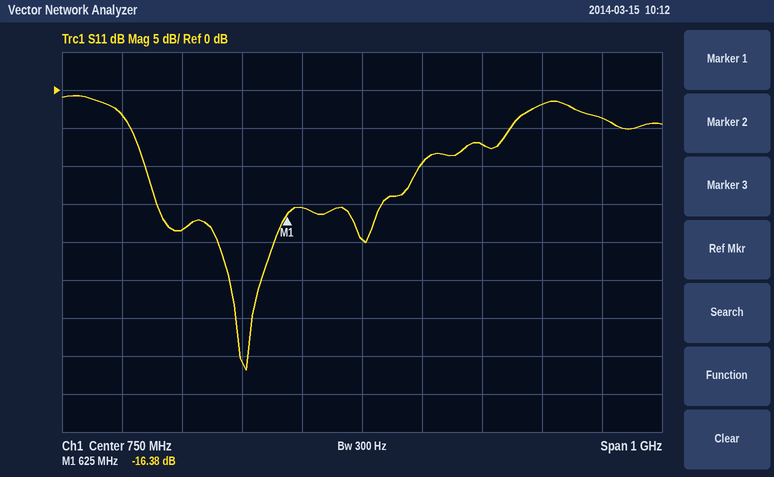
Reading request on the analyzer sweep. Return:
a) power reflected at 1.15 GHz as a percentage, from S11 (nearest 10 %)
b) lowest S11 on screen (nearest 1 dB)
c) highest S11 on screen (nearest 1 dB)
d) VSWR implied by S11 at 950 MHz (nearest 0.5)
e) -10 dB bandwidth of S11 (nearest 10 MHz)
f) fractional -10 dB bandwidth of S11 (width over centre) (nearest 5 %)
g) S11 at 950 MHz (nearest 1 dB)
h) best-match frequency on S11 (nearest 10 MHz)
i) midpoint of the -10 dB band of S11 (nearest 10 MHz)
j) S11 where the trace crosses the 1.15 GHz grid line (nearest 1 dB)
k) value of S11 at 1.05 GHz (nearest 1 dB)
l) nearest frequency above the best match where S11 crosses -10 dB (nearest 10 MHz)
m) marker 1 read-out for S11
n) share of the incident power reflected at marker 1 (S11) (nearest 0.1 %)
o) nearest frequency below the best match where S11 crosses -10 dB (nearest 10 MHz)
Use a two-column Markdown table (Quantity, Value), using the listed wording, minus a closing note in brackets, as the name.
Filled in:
| Quantity | Value |
|---|---|
| power reflected at 1.15 GHz as a percentage, from S11 | 40 % |
| lowest S11 on screen | -37 dB |
| highest S11 on screen | -1 dB |
| VSWR implied by S11 at 950 MHz | 2.5 |
| -10 dB bandwidth of S11 | 460 MHz |
| fractional -10 dB bandwidth of S11 (width over centre) | 75 % |
| S11 at 950 MHz | -7 dB |
| best-match frequency on S11 | 560 MHz |
| midpoint of the -10 dB band of S11 | 620 MHz |
| S11 where the trace crosses the 1.15 GHz grid line | -4 dB |
| value of S11 at 1.05 GHz | -2 dB |
| nearest frequency above the best match where S11 crosses -10 dB | 850 MHz |
| marker 1 read-out for S11 | -16.38 dB |
| share of the incident power reflected at marker 1 (S11) | 2.3 % |
| nearest frequency below the best match where S11 crosses -10 dB | 390 MHz |
